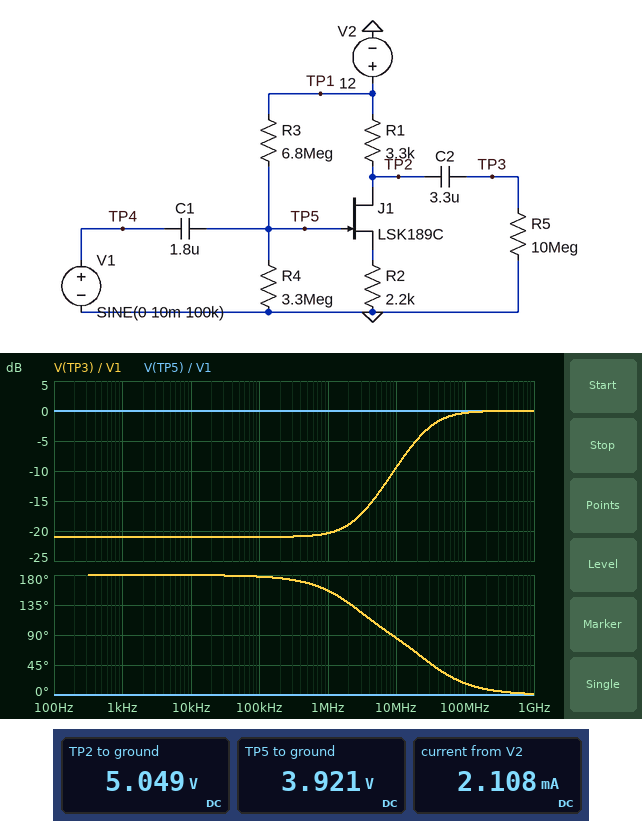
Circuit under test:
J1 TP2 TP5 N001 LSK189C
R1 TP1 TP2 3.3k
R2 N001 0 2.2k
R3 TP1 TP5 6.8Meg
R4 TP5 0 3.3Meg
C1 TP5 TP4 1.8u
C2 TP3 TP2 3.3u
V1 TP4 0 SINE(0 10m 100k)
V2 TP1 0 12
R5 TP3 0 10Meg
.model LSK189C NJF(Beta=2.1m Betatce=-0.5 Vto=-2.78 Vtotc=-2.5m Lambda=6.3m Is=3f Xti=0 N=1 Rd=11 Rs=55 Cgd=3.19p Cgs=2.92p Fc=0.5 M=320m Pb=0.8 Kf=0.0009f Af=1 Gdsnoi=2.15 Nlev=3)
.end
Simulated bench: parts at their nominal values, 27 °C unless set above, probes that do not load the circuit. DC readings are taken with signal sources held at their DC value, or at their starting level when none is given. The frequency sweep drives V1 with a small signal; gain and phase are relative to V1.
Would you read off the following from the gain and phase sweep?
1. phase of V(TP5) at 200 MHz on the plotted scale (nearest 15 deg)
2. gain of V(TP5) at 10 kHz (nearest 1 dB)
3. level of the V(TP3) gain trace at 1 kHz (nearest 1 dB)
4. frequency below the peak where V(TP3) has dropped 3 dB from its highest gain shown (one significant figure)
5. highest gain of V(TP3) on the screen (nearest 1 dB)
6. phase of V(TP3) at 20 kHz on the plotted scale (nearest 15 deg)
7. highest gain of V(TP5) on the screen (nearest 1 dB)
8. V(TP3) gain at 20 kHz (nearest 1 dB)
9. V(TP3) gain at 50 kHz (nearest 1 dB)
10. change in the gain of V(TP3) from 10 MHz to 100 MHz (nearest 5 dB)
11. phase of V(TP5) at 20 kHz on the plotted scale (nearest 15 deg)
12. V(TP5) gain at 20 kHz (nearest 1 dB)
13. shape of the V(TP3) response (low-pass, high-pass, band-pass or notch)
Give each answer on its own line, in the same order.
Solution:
0 deg
0 dB
-21 dB
30 MHz
0 dB
180 deg
0 dB
-21 dB
-21 dB
10 dB
0 deg
0 dB
high-pass
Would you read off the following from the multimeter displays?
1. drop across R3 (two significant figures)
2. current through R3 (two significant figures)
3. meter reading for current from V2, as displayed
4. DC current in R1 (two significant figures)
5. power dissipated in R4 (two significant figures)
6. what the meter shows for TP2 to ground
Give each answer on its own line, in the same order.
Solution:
8.1 V
1.2 µA
2.108 mA
2.1 mA
4.7 µW
5.049 V
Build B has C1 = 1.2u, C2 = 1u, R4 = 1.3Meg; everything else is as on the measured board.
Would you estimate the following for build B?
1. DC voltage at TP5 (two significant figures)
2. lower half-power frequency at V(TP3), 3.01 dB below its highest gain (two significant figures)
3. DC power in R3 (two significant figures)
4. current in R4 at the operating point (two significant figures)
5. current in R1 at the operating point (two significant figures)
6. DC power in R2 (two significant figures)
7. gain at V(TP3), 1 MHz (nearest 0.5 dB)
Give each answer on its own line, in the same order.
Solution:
1.9 V
120 mHz
15 µW
1.5 µA
1.7 mA
6.3 mW
2.5 dB
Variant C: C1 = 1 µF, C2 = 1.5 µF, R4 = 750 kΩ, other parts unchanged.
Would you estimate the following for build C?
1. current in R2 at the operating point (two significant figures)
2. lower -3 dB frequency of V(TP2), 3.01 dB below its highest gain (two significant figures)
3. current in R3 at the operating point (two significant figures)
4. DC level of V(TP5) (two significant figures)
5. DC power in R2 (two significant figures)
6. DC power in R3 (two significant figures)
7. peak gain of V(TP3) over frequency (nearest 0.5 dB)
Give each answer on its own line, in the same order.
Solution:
1.4 mA
240 mHz
1.6 µA
1.2 V
4.3 mW
17 µW
2.0 dB
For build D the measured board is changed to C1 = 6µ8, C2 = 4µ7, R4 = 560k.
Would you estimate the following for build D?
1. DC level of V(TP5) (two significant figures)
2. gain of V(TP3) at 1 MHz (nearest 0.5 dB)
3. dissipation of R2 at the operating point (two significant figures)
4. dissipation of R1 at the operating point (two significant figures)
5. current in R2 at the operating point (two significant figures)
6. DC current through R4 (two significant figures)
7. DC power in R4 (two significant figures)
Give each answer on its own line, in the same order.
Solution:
910 mV
2.0 dB
3.7 mW
5.5 mW
1.3 mA
1.6 µA
1.5 µW
